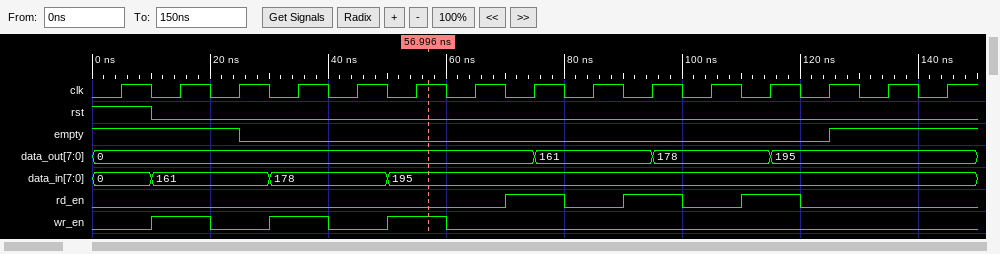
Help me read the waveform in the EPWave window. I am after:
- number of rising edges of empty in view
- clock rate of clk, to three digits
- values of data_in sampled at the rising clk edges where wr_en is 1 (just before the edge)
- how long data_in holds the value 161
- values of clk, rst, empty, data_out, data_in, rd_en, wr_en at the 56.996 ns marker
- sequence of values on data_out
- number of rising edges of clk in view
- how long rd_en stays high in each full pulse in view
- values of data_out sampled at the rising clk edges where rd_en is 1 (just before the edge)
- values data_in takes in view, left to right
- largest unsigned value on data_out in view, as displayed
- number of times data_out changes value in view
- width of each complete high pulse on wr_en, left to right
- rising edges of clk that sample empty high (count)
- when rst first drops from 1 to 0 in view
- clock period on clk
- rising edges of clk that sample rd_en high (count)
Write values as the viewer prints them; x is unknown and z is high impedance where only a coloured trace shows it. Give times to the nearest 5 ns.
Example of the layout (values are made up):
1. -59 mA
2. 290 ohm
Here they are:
1. 1
2. 100 MHz
3. 161, 178, 195
4. 20 ns
5. clk=1, rst=0, empty=0, data_out=0, data_in=195, rd_en=0, wr_en=1
6. 0, 161, 178, 195
7. 15
8. 10 ns, 10 ns, 10 ns
9. 0, 161, 178
10. 0, 161, 178, 195
11. 195
12. 3
13. 10 ns, 10 ns, 10 ns
14. 5
15. 10 ns
16. 10 ns
17. 3
